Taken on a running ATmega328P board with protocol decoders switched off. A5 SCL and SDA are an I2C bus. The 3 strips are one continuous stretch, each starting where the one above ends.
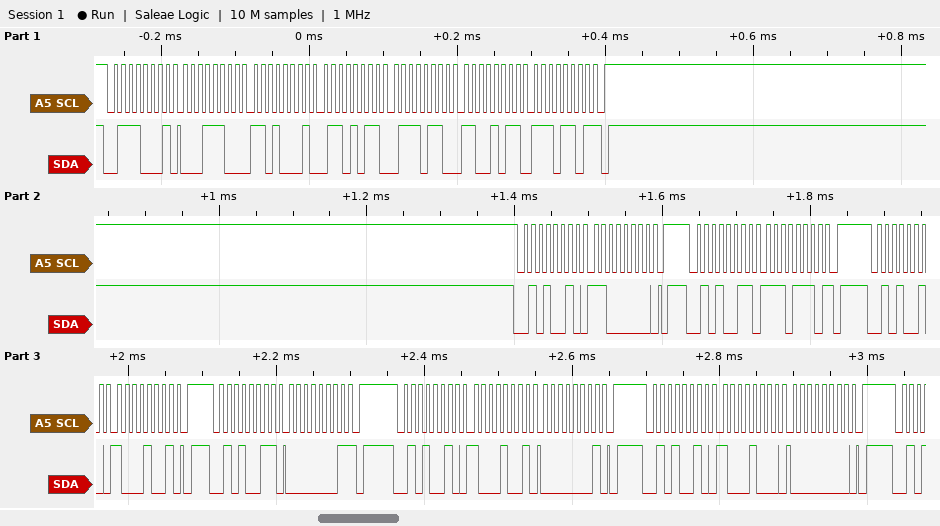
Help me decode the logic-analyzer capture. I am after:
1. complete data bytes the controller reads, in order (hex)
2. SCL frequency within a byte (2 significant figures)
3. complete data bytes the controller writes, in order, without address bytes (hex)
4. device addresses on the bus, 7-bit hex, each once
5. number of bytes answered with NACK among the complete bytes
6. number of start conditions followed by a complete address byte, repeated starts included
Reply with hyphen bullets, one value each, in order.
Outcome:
- 1C D1 6B 76 CB ED EE 01
- 100 kHz
- C0 89 89 01 88 00
- 0x38 0x29
- 3
- 7
